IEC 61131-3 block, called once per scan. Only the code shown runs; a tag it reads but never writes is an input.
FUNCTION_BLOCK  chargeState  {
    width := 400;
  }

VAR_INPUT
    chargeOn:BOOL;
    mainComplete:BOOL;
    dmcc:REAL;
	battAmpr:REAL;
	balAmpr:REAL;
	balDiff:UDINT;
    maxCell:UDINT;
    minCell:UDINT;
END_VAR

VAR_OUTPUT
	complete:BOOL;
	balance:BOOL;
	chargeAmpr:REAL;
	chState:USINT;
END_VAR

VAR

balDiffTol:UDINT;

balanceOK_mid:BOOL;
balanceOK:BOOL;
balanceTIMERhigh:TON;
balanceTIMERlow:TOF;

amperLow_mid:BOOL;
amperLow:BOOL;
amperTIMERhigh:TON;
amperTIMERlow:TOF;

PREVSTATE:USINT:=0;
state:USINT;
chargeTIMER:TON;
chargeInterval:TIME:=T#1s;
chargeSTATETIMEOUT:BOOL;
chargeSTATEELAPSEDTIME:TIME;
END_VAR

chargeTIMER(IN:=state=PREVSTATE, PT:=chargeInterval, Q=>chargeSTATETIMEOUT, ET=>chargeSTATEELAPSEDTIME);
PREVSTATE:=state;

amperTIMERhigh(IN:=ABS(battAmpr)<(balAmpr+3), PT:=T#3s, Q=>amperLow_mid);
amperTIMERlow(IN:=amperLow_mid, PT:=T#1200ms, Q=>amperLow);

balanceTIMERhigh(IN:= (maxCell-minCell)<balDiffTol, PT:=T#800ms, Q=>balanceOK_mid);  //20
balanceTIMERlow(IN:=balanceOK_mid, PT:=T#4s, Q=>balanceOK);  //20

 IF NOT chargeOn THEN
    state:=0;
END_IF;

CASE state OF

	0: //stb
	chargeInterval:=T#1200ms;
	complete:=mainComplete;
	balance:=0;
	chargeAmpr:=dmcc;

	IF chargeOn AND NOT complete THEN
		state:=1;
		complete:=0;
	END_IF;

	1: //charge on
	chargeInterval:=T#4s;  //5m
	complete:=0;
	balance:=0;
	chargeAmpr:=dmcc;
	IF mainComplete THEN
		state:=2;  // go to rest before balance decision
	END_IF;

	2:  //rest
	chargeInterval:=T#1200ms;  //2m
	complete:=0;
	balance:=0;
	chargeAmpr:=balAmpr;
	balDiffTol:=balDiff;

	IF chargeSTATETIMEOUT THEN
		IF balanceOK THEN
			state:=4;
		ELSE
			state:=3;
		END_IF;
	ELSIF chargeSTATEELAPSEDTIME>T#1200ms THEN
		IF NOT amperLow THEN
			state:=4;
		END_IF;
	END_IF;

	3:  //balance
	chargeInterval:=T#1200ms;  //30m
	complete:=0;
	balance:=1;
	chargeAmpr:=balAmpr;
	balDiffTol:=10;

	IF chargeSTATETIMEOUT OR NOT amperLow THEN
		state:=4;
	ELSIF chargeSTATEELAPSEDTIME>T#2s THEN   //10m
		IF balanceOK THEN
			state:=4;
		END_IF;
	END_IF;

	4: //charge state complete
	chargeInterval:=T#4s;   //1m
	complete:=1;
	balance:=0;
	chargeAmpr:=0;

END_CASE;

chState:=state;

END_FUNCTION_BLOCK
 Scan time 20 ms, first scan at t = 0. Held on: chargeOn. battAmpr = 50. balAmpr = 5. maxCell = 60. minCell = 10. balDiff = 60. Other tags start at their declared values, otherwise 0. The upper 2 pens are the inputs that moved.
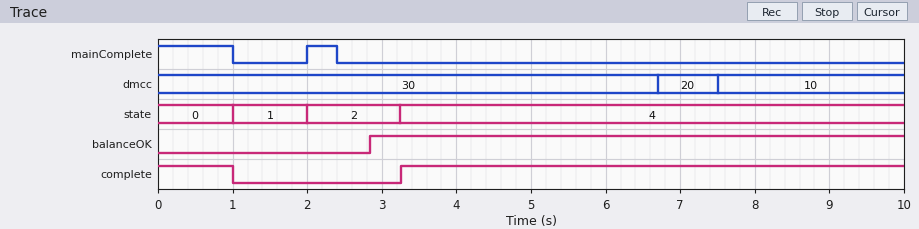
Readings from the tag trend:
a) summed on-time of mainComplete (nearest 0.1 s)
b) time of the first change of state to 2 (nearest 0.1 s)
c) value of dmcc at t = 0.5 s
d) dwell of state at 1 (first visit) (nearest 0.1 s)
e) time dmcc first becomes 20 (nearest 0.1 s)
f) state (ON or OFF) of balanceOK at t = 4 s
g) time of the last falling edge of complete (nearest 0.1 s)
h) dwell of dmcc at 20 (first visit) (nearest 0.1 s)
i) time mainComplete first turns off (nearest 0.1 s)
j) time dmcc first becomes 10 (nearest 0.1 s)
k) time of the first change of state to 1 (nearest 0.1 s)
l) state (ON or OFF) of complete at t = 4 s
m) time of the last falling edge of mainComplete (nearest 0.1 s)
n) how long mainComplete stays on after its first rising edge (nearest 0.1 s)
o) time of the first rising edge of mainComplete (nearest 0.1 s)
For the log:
1.4 s
2.0 s
30
1.0 s
6.7 s
ON
1.0 s
0.8 s
1.0 s
7.5 s
1.0 s
ON
2.4 s
0.4 s
2.0 s
